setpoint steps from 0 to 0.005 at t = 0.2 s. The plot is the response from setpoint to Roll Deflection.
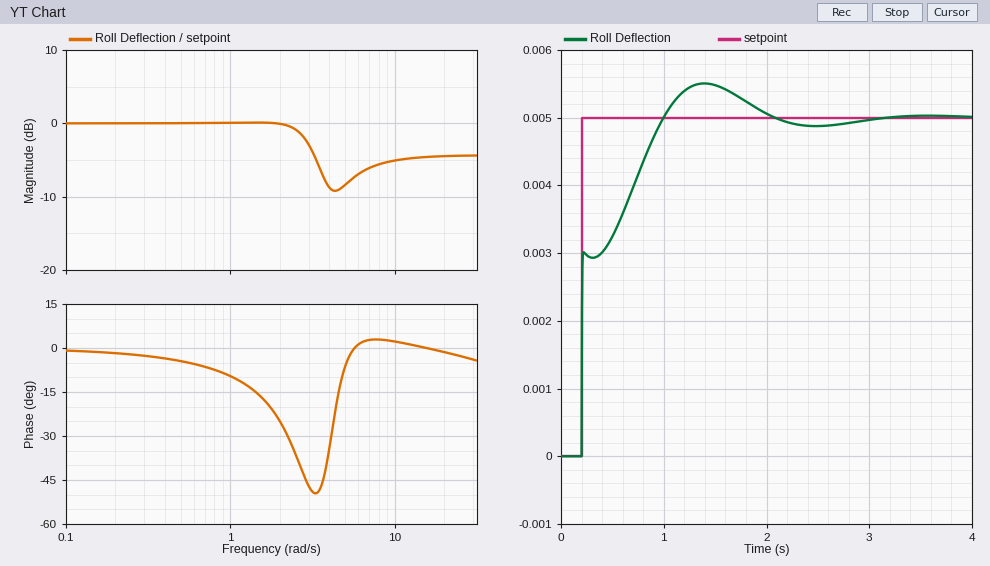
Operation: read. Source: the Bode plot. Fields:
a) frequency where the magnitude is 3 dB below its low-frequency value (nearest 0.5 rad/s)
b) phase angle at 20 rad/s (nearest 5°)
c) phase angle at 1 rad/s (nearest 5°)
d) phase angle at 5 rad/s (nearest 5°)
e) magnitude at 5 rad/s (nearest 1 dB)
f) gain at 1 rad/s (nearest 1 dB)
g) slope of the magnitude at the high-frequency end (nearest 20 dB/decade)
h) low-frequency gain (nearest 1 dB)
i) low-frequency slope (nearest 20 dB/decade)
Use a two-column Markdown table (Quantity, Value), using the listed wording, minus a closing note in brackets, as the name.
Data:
| Quantity | Value |
|---|---|
| frequency where the magnitude is 3 dB below its low-frequency value | 3.0 rad/s |
| phase angle at 20 rad/s | 0° |
| phase angle at 1 rad/s | -10° |
| phase angle at 5 rad/s | -5° |
| magnitude at 5 rad/s | -8 dB |
| gain at 1 rad/s | 0 dB |
| slope of the magnitude at the high-frequency end | 0 dB/decade |
| low-frequency gain | 0 dB |
| low-frequency slope | 0 dB/decade |
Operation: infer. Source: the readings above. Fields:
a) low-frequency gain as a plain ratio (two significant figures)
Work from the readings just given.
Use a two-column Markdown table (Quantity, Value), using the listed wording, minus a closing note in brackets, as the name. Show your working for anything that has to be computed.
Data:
| Quantity | Value |
|---|---|
| low-frequency gain as a plain ratio | 10^(0 / 20) = 1.0 |
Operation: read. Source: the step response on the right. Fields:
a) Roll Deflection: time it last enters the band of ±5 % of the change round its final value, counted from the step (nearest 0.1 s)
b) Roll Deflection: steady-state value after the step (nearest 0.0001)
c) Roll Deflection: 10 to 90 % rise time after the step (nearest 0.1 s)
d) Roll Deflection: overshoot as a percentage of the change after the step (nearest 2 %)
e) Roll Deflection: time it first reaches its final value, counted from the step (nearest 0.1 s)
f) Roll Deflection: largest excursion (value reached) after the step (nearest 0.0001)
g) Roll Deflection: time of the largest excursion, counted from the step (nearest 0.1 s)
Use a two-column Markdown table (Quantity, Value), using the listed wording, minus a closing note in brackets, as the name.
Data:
| Quantity | Value |
|---|---|
| Roll Deflection: time it last enters the band of ±5 % of the change round its final value, counted from the step | 1.6 s |
| Roll Deflection: steady-state value after the step | 0.0050 |
| Roll Deflection: 10 to 90 % rise time after the step | 0.6 s |
| Roll Deflection: overshoot as a percentage of the change after the step | 10 % |
| Roll Deflection: time it first reaches its final value, counted from the step | 0.8 s |
| Roll Deflection: largest excursion (value reached) after the step | 0.0055 |
| Roll Deflection: time of the largest excursion, counted from the step | 1.2 s |
